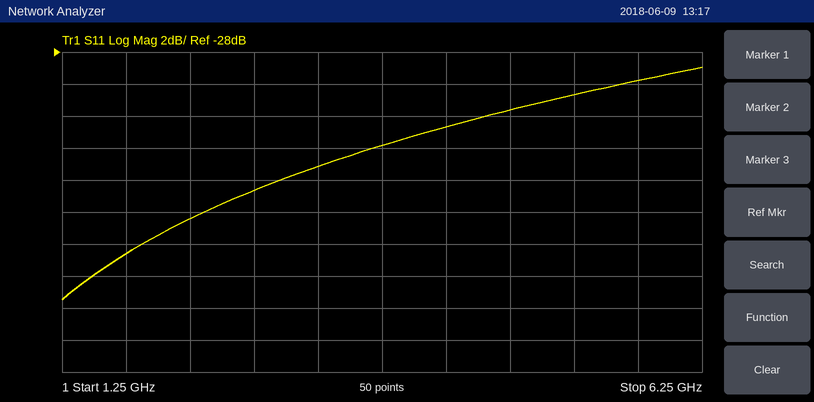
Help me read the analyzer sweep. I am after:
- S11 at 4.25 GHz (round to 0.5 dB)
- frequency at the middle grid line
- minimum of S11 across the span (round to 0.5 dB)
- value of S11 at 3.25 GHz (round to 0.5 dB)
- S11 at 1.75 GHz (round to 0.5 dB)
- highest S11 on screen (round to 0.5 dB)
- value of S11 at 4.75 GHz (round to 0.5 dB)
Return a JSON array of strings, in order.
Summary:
["-32.5 dB", "3.75 GHz", "-43.5 dB", "-35.0 dB", "-40.5 dB", "-29.0 dB", "-31.5 dB"]
